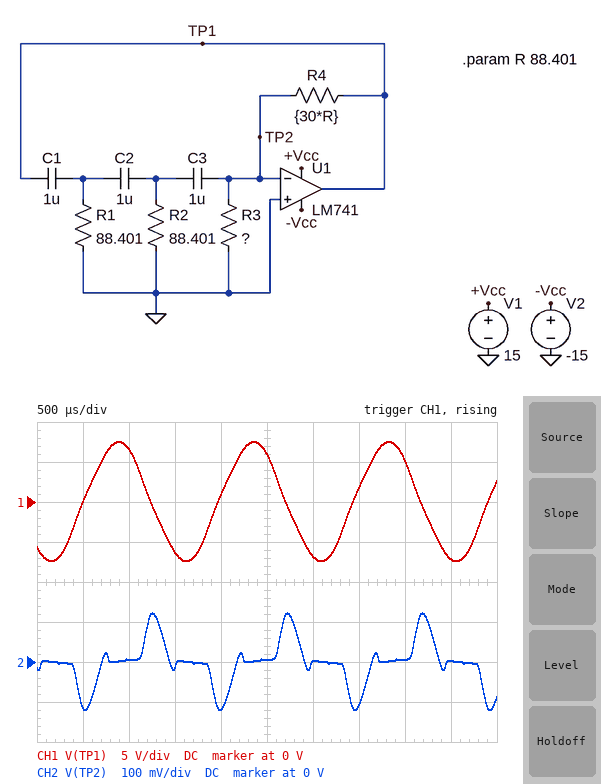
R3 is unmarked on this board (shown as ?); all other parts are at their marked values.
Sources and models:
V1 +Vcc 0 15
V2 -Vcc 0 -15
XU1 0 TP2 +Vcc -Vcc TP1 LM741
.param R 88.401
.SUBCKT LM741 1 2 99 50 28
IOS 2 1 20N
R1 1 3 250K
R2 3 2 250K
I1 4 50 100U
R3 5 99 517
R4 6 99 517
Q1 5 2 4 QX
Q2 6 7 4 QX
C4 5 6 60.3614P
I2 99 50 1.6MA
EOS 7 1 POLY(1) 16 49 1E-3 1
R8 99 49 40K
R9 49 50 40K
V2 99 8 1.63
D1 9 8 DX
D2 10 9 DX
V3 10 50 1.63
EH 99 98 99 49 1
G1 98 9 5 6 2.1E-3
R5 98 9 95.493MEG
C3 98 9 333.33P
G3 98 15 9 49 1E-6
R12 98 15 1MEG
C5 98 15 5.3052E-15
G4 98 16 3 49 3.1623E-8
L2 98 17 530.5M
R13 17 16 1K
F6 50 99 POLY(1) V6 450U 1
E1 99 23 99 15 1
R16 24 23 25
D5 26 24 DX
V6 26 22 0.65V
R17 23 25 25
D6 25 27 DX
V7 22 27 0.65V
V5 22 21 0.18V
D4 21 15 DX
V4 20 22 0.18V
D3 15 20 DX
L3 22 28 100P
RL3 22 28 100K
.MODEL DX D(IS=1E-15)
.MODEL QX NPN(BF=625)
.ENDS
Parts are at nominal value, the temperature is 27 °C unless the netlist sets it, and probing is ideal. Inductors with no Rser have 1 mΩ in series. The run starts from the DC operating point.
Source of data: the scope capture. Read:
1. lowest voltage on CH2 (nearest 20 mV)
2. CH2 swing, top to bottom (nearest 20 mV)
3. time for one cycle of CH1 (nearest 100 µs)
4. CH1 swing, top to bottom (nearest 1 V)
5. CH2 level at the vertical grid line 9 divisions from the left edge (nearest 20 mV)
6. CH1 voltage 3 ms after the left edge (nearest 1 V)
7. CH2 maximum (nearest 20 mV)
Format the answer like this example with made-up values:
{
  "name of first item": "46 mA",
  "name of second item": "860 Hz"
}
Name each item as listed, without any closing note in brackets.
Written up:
{
  "lowest voltage on CH2": "-120 mV",
  "CH2 swing, top to bottom": "240 mV",
  "time for one cycle of CH1": "1.5 ms",
  "CH1 swing, top to bottom": "15 V",
  "CH2 level at the vertical grid line 9 divisions from the left edge": "0 V",
  "CH1 voltage 3 ms after the left edge": "-7 V",
  "CH2 maximum": "120 mV"
}
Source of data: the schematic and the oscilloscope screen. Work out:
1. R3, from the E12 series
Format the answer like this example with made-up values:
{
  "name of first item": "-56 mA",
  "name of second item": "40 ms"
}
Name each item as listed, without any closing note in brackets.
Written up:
{
  "R3, from the E12 series": "68 Ω"
}
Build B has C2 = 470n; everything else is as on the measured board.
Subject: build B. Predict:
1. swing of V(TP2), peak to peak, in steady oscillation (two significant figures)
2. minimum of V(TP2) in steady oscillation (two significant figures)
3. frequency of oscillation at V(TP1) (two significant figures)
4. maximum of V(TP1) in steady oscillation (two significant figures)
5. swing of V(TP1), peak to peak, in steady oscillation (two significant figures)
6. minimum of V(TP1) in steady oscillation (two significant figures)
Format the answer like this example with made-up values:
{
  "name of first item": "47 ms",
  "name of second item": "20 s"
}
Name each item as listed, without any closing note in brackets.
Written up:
{
  "swing of V(TP2), peak to peak, in steady oscillation": "210 mV",
  "minimum of V(TP2) in steady oscillation": "-100 mV",
  "frequency of oscillation at V(TP1)": "850 Hz",
  "maximum of V(TP1) in steady oscillation": "6.2 V",
  "swing of V(TP1), peak to peak, in steady oscillation": "12 V",
  "minimum of V(TP1) in steady oscillation": "-6.1 V"
}
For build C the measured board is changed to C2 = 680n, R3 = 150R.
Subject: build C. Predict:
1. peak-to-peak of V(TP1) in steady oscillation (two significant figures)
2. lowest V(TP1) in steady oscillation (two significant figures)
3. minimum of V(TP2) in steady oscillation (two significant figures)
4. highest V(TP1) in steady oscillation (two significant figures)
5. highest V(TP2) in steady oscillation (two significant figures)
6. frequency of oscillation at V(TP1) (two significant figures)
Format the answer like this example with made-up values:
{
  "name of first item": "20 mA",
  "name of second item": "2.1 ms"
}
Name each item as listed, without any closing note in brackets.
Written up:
{
  "peak-to-peak of V(TP1) in steady oscillation": "14 V",
  "lowest V(TP1) in steady oscillation": "-7.0 V",
  "minimum of V(TP2) in steady oscillation": "-200 mV",
  "highest V(TP1) in steady oscillation": "7.0 V",
  "highest V(TP2) in steady oscillation": "200 mV",
  "frequency of oscillation at V(TP1)": "750 Hz"
}
